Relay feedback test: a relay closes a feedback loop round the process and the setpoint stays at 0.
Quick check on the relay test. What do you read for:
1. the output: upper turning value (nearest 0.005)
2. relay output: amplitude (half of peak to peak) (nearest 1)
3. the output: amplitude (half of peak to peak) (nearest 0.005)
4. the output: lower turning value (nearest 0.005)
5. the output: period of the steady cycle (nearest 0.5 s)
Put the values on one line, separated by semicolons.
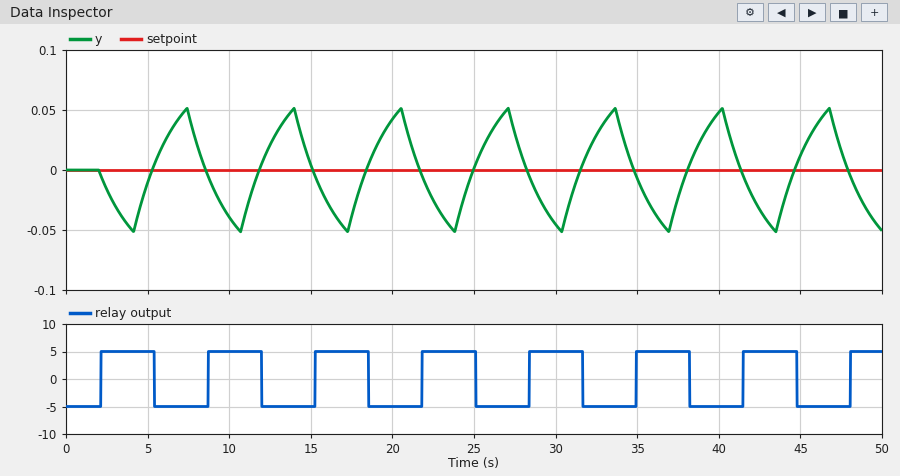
0.050; 5; 0.050; -0.050; 6.5 s
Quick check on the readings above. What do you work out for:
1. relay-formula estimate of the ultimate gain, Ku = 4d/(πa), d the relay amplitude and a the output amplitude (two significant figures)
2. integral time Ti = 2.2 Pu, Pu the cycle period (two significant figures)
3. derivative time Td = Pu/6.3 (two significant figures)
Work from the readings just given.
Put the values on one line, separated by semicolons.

130; 14 s; 1.0 s
